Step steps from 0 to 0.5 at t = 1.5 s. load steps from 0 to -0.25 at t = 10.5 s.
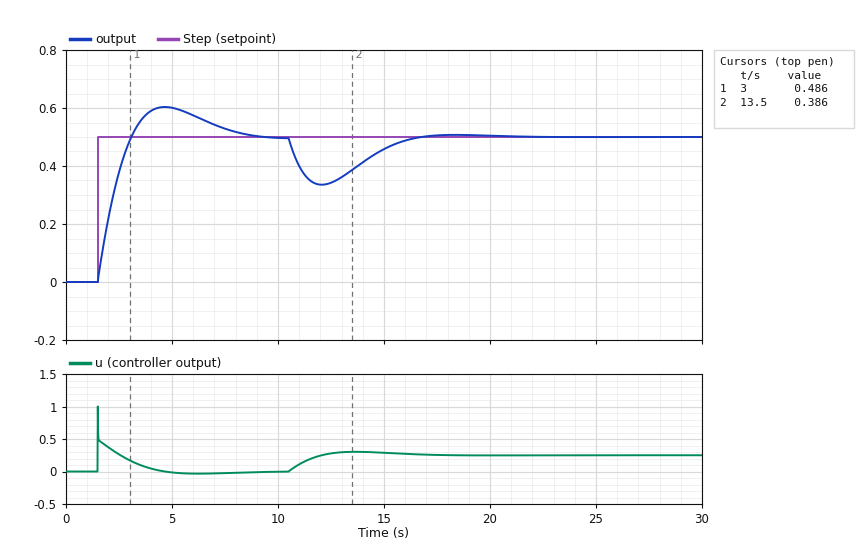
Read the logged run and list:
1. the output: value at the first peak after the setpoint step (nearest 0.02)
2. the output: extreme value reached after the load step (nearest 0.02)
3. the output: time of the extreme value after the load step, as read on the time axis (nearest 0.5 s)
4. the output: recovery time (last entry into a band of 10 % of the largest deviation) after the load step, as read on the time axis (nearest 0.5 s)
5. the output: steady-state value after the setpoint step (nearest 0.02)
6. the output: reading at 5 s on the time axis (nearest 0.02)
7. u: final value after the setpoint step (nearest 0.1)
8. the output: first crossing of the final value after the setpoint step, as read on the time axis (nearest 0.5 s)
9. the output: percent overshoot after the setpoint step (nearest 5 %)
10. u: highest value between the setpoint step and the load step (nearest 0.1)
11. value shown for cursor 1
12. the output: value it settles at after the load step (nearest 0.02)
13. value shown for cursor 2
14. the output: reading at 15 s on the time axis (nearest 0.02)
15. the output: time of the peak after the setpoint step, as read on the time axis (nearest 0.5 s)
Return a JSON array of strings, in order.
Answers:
["0.60", "0.34", "12.0 s", "16.0 s", "0.50", "0.60", "0.0", "3.0 s", "20 %", "1.0", "0.486", "0.50", "0.386", "0.46", "4.5 s"]
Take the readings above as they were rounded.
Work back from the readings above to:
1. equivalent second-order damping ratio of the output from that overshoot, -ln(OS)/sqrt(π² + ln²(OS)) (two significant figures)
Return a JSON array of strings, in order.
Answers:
["0.46"]
